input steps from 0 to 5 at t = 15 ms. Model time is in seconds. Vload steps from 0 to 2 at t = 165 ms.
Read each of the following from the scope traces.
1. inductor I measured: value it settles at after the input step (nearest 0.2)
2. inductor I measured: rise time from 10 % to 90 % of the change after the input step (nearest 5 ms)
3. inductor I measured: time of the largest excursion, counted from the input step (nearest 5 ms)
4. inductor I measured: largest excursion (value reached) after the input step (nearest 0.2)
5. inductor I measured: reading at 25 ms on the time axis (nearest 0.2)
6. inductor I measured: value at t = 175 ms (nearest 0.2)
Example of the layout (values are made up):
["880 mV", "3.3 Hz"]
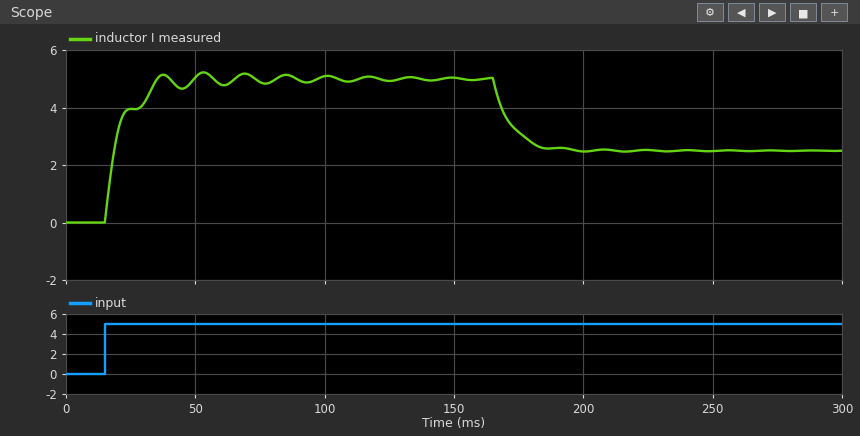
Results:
["5.0", "15 ms", "40 ms", "5.2", "4.0", "3.2"]
